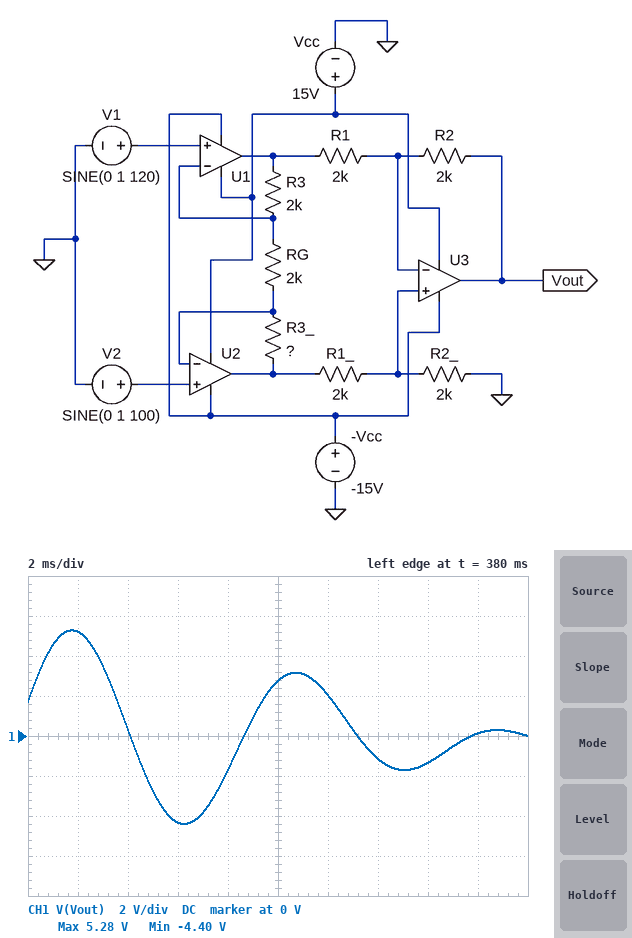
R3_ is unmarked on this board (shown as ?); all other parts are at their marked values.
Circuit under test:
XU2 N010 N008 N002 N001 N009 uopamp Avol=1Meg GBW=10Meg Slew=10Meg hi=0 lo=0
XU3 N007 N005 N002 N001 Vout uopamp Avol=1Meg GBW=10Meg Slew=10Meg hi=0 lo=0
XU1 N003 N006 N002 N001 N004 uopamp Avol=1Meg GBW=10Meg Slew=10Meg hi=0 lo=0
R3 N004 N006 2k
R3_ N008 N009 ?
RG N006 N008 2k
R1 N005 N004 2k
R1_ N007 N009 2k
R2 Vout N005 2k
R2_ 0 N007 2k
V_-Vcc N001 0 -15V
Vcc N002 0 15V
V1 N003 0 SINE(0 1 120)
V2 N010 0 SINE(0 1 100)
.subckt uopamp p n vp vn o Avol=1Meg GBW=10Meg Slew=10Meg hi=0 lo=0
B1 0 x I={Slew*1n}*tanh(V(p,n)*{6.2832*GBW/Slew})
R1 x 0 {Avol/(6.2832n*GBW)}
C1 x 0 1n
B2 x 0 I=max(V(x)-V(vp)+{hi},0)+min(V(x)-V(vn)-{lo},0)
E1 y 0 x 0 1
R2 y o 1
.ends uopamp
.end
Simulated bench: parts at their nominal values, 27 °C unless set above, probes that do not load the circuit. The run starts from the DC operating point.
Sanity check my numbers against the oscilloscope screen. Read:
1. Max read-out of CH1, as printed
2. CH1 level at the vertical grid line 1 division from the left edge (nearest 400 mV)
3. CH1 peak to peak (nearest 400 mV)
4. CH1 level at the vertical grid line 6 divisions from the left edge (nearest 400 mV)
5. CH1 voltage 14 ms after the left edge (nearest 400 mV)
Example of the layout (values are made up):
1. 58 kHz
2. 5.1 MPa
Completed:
1. 5.28 V
2. 5.2 V
3. 9.6 V
4. 2.0 V
5. -1.2 V
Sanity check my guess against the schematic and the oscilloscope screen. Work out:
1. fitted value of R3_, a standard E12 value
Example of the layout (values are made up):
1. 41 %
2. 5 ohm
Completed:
1. 1.8 kΩ
